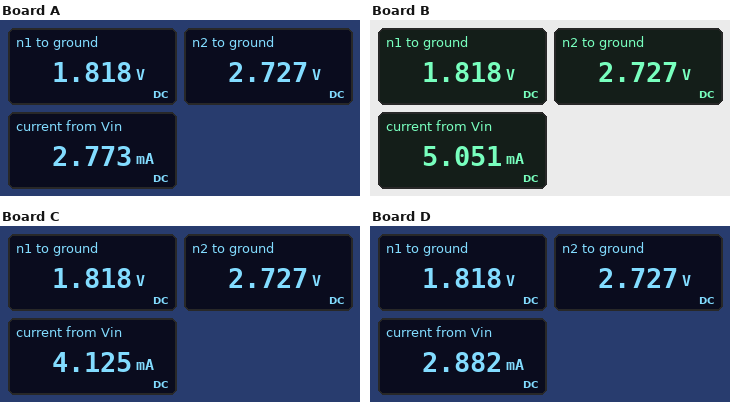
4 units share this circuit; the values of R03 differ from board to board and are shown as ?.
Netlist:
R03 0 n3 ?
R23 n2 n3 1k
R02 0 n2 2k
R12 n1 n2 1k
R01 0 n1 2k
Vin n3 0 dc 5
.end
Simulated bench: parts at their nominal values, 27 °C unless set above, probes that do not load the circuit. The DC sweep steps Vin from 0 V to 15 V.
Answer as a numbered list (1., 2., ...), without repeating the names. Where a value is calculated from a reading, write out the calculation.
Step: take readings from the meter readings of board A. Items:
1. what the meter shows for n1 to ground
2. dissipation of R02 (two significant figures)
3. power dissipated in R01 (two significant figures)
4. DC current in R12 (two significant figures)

1. 1.818 V
2. (2.727 V)^2 / 2 kΩ = 3.7 mW
3. (1.818 V)^2 / 2 kΩ = 1.7 mW
4. (2.727 V - 1.818 V) / 1 kΩ = 910 µA
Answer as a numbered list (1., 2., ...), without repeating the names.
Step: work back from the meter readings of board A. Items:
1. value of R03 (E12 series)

1. 10 kΩ
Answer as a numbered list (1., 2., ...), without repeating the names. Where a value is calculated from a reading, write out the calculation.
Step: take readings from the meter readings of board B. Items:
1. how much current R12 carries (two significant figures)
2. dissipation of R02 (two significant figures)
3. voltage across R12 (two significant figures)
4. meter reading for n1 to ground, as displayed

1. (2.727 V - 1.818 V) / 1 kΩ = 910 µA
2. (2.727 V)^2 / 2 kΩ = 3.7 mW
3. 2.727 V - 1.818 V = 910 mV
4. 1.818 V
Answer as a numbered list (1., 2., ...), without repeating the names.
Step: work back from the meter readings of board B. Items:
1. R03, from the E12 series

1. 1.8 kΩ
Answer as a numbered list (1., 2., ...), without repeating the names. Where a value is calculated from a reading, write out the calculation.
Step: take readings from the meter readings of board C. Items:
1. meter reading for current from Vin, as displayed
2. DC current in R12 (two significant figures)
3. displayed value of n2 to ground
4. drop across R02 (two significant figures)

1. 4.125 mA
2. (2.727 V - 1.818 V) / 1 kΩ = 910 µA
3. 2.727 V
4. 2.727 V = 2.7 V
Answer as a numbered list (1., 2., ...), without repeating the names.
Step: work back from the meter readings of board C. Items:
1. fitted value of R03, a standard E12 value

1. 2.7 kΩ
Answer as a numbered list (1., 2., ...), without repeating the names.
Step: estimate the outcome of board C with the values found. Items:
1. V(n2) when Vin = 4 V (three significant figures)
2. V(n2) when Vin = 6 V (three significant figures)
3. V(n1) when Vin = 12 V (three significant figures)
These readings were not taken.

1. 2.18 V
2. 3.27 V
3. 4.36 V
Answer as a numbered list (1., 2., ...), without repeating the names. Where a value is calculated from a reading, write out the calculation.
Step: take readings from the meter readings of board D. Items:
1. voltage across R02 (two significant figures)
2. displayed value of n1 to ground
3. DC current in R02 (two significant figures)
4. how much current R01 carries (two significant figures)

1. 2.727 V = 2.7 V
2. 1.818 V
3. (2.727 V) / 2 kΩ = 1.4 mA
4. (1.818 V) / 2 kΩ = 910 µA
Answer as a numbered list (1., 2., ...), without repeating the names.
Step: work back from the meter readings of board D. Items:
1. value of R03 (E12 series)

1. 8.2 kΩ
